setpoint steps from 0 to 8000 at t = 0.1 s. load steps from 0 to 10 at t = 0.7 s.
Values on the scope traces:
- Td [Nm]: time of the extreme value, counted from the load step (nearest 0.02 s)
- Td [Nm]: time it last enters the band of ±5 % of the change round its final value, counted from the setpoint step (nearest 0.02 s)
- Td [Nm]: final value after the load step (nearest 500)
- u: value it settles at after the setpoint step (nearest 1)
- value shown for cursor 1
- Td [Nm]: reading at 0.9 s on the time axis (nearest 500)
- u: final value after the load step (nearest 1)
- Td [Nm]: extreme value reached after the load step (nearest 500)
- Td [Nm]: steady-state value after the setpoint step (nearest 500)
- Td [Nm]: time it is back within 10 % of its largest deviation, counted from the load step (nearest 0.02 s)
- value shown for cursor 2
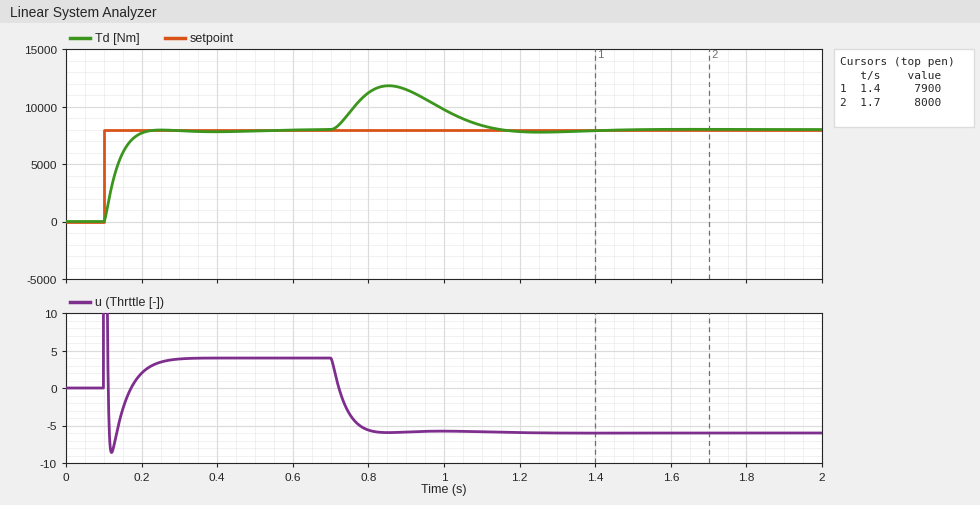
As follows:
0.16 s
0.10 s
8000
4
7900
11500
-6
12000
8000
0.40 s
8000
